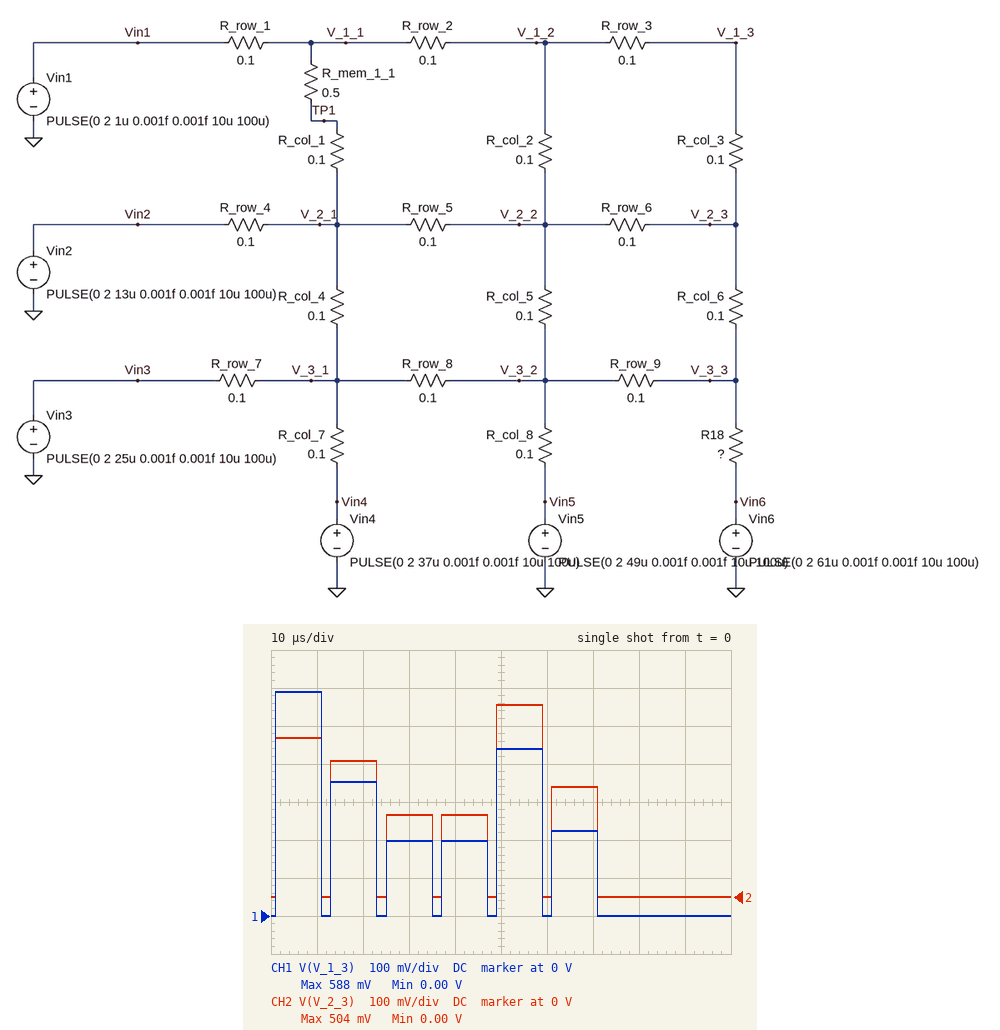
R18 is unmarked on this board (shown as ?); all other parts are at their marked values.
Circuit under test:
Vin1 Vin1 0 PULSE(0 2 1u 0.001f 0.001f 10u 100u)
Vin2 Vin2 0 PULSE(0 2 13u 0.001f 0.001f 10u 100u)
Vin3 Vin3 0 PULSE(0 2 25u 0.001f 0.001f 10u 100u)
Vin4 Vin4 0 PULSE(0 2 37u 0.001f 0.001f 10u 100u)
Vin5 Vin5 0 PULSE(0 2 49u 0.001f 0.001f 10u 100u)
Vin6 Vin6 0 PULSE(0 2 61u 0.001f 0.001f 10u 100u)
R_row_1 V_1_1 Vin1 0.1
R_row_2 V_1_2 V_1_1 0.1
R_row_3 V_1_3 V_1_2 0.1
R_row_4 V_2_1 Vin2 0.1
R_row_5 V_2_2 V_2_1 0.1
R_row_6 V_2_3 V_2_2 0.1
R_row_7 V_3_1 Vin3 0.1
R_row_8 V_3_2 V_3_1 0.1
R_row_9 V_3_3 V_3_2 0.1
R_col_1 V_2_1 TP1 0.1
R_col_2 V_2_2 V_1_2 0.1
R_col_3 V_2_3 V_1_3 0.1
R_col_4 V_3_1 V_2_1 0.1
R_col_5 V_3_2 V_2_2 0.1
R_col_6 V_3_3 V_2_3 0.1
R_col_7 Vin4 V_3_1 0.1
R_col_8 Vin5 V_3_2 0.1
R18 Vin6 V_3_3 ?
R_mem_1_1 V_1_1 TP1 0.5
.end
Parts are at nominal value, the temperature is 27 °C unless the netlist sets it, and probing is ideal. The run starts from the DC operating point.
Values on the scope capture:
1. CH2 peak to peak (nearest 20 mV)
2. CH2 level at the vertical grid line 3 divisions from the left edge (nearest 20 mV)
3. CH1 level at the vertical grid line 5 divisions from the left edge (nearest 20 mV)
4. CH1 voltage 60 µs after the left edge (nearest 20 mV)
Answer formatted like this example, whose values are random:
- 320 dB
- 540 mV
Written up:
- 500 mV
- 220 mV
- 440 mV
- 0 V
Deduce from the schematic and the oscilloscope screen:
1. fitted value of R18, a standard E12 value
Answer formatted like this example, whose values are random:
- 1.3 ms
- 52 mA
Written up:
- 0.33 Ω
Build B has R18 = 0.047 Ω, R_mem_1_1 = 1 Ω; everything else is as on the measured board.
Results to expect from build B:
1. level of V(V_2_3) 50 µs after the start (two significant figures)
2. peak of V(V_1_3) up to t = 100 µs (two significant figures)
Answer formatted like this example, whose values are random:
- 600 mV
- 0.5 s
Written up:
- 290 mV
- 660 mV
